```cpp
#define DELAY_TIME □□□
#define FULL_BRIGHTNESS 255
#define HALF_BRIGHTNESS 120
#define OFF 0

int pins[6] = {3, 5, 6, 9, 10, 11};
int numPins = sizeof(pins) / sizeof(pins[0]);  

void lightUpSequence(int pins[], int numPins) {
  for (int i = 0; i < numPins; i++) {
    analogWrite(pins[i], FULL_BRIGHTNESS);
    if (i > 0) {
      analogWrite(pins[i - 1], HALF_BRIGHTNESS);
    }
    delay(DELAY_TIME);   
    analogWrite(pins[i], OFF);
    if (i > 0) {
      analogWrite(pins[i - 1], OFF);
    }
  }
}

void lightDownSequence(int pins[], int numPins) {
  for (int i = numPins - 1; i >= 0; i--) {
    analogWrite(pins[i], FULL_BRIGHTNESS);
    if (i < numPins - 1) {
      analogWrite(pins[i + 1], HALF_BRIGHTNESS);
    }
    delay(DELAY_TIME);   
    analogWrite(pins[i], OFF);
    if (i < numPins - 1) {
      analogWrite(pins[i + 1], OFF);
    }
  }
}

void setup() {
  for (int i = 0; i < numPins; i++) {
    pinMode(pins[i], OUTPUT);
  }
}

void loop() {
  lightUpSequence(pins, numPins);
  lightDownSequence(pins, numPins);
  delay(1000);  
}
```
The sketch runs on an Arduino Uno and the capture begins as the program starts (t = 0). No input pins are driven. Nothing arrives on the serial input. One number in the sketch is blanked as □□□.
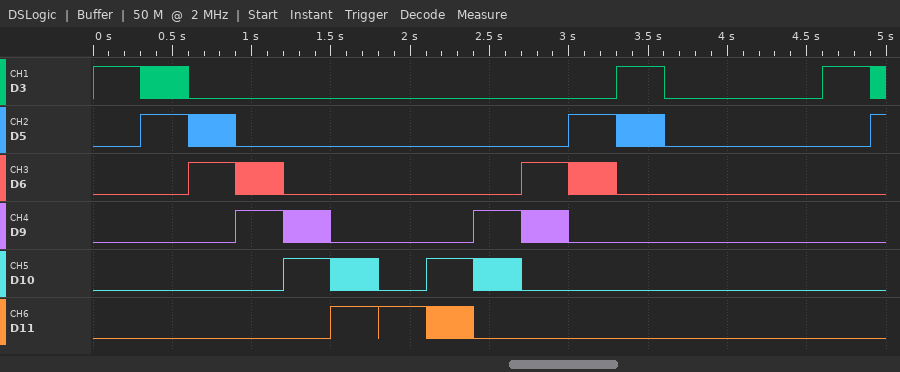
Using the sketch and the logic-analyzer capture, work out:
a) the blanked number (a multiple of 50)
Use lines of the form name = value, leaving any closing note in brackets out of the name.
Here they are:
the blanked number = 300
